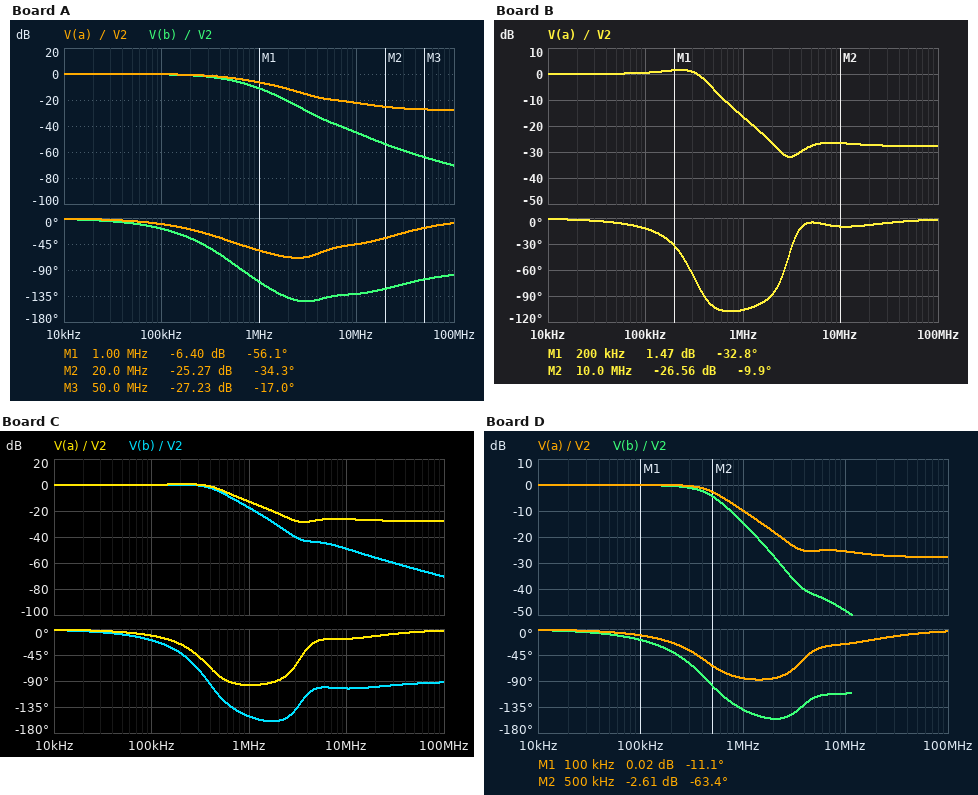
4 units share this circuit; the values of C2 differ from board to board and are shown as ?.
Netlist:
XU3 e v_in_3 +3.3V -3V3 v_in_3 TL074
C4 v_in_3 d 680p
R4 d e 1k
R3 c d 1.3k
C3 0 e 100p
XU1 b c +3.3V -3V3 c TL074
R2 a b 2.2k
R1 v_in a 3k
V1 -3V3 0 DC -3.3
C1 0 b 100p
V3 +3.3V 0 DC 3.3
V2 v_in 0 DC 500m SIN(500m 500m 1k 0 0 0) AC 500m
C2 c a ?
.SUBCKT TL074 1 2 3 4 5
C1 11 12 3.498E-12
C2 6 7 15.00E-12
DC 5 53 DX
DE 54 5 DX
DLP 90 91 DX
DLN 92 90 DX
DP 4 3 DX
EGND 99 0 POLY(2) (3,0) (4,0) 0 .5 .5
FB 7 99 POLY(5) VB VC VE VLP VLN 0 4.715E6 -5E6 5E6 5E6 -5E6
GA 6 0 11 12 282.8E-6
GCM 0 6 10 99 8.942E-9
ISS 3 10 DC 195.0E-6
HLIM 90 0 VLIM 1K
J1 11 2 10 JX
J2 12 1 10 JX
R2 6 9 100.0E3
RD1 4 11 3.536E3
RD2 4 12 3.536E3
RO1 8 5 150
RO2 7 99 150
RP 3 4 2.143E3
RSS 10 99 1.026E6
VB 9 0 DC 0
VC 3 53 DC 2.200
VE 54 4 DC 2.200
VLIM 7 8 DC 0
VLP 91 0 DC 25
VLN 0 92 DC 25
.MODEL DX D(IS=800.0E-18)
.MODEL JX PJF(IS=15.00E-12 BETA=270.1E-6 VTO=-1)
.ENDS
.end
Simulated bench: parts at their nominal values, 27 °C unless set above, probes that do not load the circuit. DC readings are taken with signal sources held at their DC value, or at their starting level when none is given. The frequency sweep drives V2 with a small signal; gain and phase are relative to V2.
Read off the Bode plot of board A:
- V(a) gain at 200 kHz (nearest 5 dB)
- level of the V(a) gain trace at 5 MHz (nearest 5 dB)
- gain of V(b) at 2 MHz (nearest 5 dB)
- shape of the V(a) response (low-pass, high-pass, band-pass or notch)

0 dB
-20 dB
-20 dB
low-pass
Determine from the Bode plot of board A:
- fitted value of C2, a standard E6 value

68 pF
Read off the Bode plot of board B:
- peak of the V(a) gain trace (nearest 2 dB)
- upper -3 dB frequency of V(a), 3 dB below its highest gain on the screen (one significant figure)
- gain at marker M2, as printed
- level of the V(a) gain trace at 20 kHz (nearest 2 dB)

2 dB
400 kHz
-26.56 dB
0 dB
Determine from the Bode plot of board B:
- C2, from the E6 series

330 pF
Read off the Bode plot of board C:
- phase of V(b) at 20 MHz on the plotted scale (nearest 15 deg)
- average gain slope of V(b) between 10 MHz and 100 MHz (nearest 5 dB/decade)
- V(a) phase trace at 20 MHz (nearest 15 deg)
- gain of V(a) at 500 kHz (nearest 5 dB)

-105 deg
-20 dB/decade
-15 deg
-5 dB
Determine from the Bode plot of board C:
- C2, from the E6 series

220 pF
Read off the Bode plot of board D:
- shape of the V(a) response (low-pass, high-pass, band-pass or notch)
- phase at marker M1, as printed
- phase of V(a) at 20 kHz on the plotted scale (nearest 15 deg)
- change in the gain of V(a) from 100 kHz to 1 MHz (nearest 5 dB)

low-pass
-11.1 deg
0 deg
-10 dB
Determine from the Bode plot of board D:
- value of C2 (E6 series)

150 pF
